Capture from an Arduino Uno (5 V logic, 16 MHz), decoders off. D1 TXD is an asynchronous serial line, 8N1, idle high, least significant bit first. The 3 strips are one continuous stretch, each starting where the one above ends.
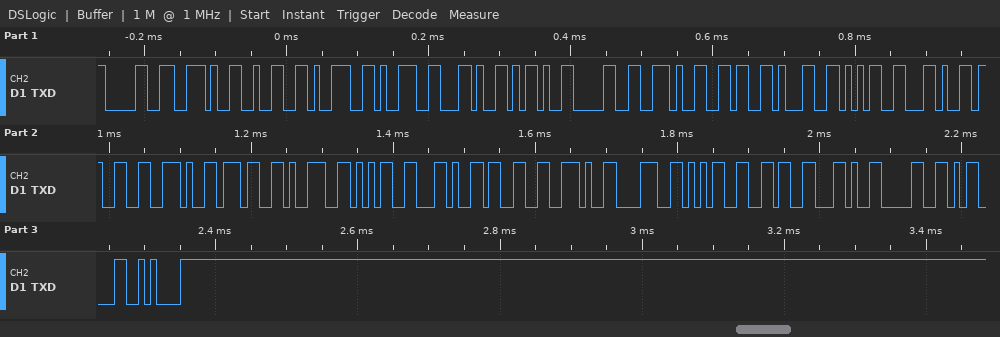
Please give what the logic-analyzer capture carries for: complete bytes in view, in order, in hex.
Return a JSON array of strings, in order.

["30 2E 32 39 39 2C 2D 30 2E 36 31 35 2C 33 2E 37 39 35 2C 33 2E 38 35 36 2C 30 0D 0A"]
